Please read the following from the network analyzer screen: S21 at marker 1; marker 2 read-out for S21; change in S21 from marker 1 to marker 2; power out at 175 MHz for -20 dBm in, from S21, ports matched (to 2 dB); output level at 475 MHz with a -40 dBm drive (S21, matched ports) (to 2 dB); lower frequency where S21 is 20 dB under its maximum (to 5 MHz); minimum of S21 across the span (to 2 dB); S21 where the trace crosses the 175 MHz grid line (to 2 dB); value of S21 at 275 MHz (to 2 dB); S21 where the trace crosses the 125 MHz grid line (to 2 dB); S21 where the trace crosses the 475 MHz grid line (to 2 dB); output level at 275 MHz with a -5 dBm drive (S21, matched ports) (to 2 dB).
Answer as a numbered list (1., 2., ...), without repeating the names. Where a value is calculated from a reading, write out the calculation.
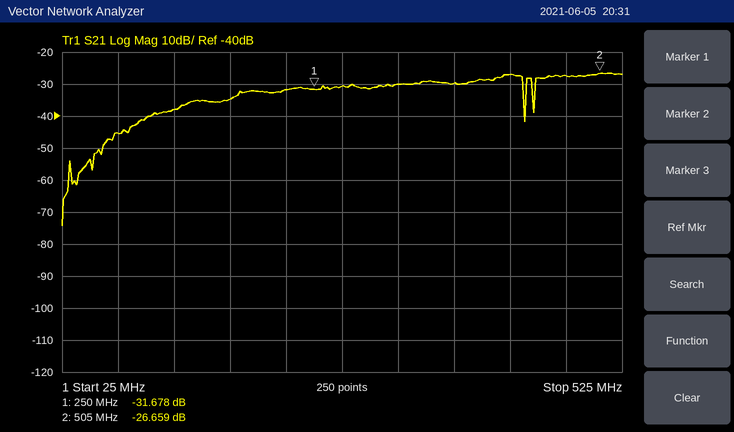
1. -31.678 dB
2. -26.659 dB
3. -26.659 − (-31.678) = 5.019 dB
4. -20 dBm + (-34 dB) = -54 dBm
5. -40 dBm + (-28 dB) = -68 dBm
6. 70 MHz
7. -74 dB
8. -34 dB
9. -30 dB
10. -38 dB
11. -28 dB
12. -5 dBm + (-30 dB) = -36 dBm
